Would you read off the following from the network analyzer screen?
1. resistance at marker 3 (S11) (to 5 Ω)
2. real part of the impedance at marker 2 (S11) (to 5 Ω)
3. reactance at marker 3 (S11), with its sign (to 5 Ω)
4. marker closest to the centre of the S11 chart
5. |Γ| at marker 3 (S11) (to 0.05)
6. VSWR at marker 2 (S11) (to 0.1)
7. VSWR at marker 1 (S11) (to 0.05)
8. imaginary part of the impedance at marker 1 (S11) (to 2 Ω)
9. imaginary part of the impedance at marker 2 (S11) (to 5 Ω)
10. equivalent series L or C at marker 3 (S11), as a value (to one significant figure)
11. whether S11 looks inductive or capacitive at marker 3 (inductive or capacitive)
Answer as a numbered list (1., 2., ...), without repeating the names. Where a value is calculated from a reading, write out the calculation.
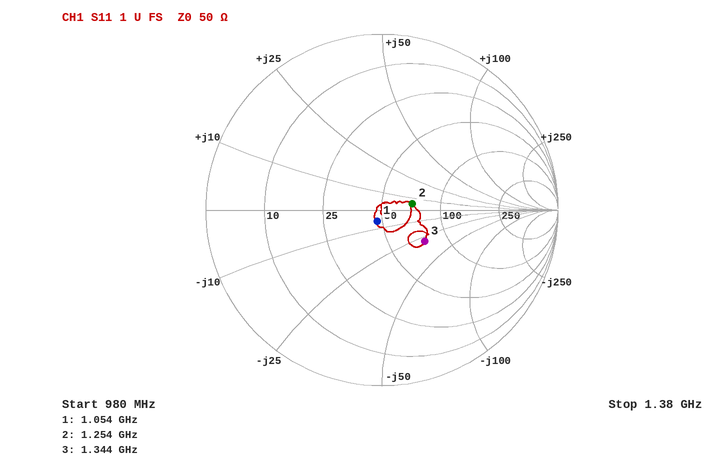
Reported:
1. 75 Ω
2. 70 Ω
3. -30 Ω
4. marker 1
5. 0.30
6. 1.4
7. 1.15
8. -6 Ω
9. +5 Ω
10. C = 1/(2π × 1.344 GHz × 30 Ω) ≈ 4 pF
11. capacitive
